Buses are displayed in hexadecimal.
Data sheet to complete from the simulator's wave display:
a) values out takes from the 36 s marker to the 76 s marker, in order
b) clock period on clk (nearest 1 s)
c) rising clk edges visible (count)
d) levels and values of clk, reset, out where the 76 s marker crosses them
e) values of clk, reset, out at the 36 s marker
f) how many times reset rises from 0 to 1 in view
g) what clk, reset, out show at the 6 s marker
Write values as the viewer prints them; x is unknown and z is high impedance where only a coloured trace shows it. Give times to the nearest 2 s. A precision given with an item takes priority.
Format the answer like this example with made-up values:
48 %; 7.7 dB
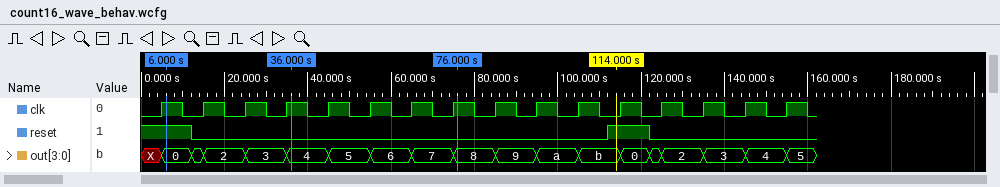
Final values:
4, 5, 6, 7, 8; 10 s; 16; clk=1, reset=0, out=8; clk=1, reset=0, out=4; 1; clk=1, reset=1, out=0
